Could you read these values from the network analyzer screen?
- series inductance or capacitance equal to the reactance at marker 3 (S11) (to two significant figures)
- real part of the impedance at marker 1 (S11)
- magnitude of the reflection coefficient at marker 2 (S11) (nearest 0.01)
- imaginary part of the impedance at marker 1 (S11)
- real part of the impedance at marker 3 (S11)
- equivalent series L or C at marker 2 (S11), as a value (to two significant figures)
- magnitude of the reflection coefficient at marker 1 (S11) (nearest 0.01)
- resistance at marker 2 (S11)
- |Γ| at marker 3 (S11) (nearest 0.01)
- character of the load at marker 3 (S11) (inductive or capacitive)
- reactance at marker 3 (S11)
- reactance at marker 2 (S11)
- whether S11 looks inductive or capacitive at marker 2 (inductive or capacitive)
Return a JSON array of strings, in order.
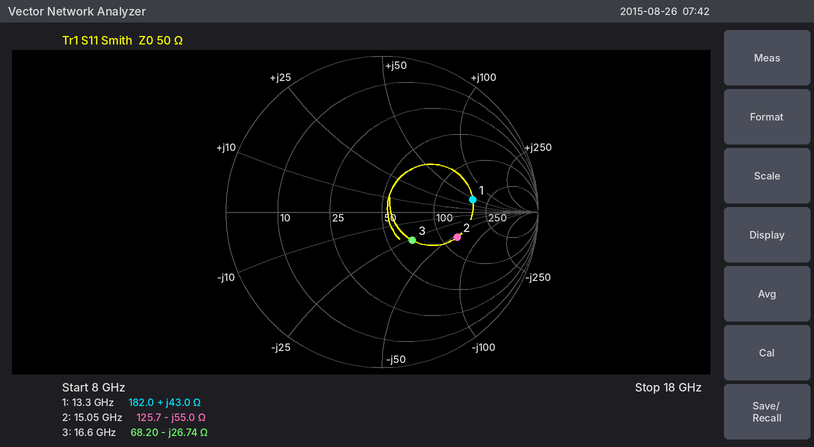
["360 fF", "182.0 Ω", "0.51", "+43.0 Ω", "68.20 Ω", "190 fF", "0.59", "125.7 Ω", "0.27", "capacitive", "-26.74 Ω", "-55.0 Ω", "capacitive"]
